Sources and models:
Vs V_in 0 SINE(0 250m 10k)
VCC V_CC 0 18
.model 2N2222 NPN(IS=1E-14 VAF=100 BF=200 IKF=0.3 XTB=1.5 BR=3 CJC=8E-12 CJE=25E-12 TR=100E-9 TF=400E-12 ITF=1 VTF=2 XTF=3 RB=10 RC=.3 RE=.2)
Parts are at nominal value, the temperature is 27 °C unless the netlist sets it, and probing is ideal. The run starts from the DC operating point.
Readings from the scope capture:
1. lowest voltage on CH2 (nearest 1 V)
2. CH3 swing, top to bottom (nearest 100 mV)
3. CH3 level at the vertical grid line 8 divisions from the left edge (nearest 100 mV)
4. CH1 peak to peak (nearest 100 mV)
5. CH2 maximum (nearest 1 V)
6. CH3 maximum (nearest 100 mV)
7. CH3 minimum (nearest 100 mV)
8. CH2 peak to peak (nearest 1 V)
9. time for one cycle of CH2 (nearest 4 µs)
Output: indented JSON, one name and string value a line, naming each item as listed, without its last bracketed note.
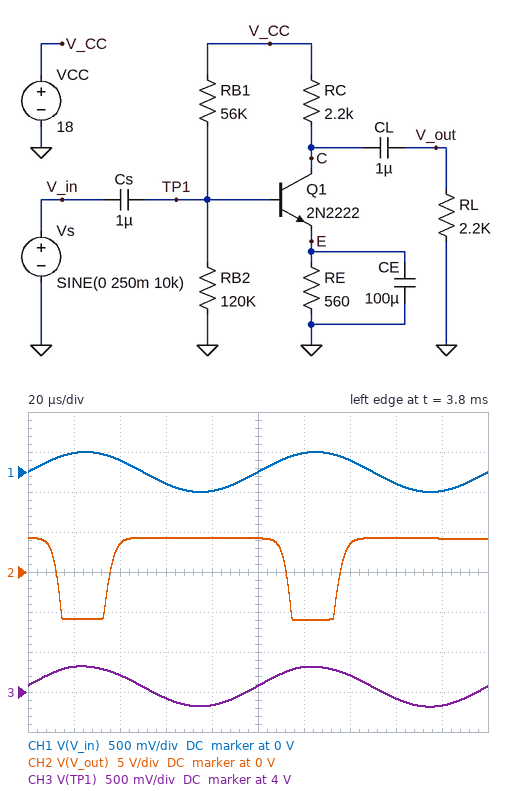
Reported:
{
  "lowest voltage on CH2": "-6 V",
  "CH3 swing, top to bottom": "500 mV",
  "CH3 level at the vertical grid line 8 divisions from the left edge": "3.9 V",
  "CH1 peak to peak": "500 mV",
  "CH2 maximum": "4 V",
  "CH3 maximum": "4.3 V",
  "CH3 minimum": "3.8 V",
  "CH2 peak to peak": "10 V",
  "time for one cycle of CH2": "100 µs"
}
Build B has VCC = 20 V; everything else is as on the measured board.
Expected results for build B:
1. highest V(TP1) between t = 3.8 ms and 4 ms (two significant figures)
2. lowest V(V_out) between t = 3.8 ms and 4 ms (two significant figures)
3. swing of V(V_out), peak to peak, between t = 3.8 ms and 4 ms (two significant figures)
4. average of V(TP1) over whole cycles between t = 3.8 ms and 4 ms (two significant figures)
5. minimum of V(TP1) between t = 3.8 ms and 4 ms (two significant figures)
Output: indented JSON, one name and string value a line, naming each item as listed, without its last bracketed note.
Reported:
{
  "highest V(TP1) between t = 3.8 ms and 4 ms": "4.7 V",
  "lowest V(V_out) between t = 3.8 ms and 4 ms": "-6.6 V",
  "swing of V(V_out), peak to peak, between t = 3.8 ms and 4 ms": "11 V",
  "average of V(TP1) over whole cycles between t = 3.8 ms and 4 ms": "4.5 V",
  "minimum of V(TP1) between t = 3.8 ms and 4 ms": "4.2 V"
}
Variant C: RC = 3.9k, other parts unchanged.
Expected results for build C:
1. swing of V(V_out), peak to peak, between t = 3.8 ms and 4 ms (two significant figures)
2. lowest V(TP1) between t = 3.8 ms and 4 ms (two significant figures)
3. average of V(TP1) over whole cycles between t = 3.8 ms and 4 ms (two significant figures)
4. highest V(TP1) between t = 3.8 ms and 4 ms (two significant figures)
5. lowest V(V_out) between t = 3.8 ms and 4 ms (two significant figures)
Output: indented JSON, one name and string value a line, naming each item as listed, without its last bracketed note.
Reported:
{
  "swing of V(V_out), peak to peak, between t = 3.8 ms and 4 ms": "8.9 V",
  "lowest V(TP1) between t = 3.8 ms and 4 ms": "2.5 V",
  "average of V(TP1) over whole cycles between t = 3.8 ms and 4 ms": "2.8 V",
  "highest V(TP1) between t = 3.8 ms and 4 ms": "3.0 V",
  "lowest V(V_out) between t = 3.8 ms and 4 ms": "-5.0 V"
}
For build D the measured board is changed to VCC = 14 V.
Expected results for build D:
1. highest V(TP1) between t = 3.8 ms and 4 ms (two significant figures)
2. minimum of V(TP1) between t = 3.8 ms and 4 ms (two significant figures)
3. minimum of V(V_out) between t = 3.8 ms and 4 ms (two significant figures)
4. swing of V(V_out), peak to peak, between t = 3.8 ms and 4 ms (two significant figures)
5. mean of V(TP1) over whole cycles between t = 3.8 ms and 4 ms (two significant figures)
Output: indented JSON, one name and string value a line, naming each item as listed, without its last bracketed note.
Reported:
{
  "highest V(TP1) between t = 3.8 ms and 4 ms": "3.5 V",
  "minimum of V(TP1) between t = 3.8 ms and 4 ms": "3.0 V",
  "minimum of V(V_out) between t = 3.8 ms and 4 ms": "-4.7 V",
  "swing of V(V_out), peak to peak, between t = 3.8 ms and 4 ms": "8.0 V",
  "mean of V(TP1) over whole cycles between t = 3.8 ms and 4 ms": "3.3 V"
}
